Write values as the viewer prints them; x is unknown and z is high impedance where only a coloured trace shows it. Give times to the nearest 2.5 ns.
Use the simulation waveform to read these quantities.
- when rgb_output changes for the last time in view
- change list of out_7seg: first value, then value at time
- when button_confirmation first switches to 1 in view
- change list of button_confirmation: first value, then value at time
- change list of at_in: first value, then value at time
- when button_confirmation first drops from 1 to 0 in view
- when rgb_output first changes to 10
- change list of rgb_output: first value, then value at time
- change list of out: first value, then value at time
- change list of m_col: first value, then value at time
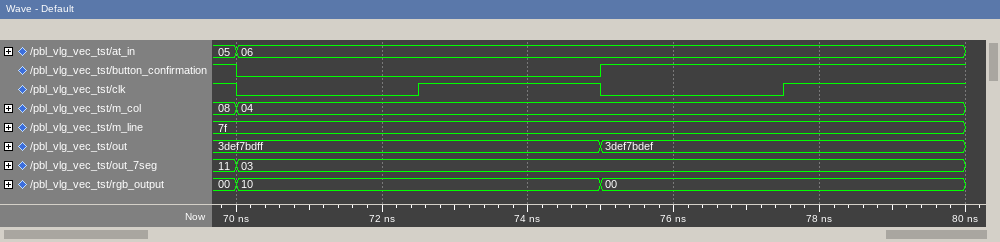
75 ns
11, 03 at 70 ns
75 ns
1, 0 at 70 ns, 1 at 75 ns
05, 06 at 70 ns
70 ns
70 ns
00, 10 at 70 ns, 00 at 75 ns
3def7bdff, 3def7bdef at 75 ns
08, 04 at 70 ns
